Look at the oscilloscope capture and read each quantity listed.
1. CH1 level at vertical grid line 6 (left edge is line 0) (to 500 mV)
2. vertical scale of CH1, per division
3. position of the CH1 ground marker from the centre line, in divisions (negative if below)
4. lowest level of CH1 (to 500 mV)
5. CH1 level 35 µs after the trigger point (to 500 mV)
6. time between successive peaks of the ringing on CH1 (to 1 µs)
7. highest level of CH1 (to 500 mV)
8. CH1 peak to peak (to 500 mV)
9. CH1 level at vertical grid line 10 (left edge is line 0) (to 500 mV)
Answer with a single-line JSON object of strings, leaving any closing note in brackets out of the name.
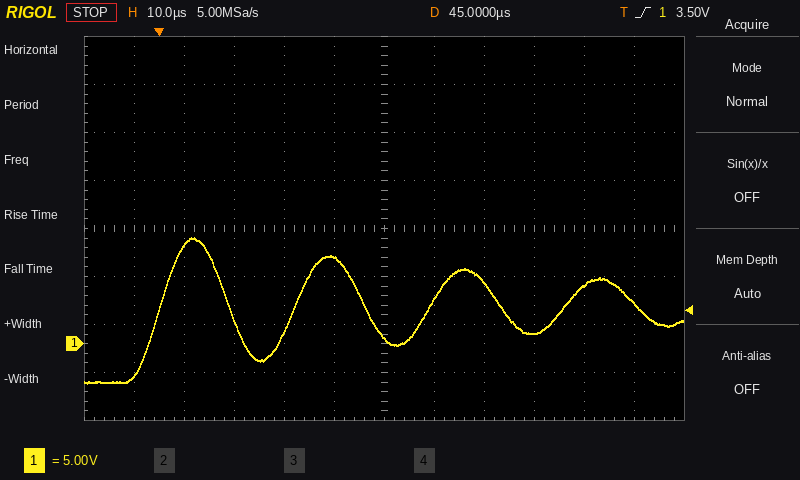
{"CH1 level at vertical grid line 6 (left edge is line 0)": "500 mV", "vertical scale of CH1, per division": "5 V", "position of the CH1 ground marker from the centre line, in divisions": "-2.4 div", "lowest level of CH1": "-4.0 V", "CH1 level 35 µs after the trigger point": "9.0 V", "time between successive peaks of the ringing on CH1": "27 µs", "highest level of CH1": "11.0 V", "CH1 peak to peak": "15.0 V", "CH1 level at vertical grid line 10 (left edge is line 0)": "6.0 V"}
